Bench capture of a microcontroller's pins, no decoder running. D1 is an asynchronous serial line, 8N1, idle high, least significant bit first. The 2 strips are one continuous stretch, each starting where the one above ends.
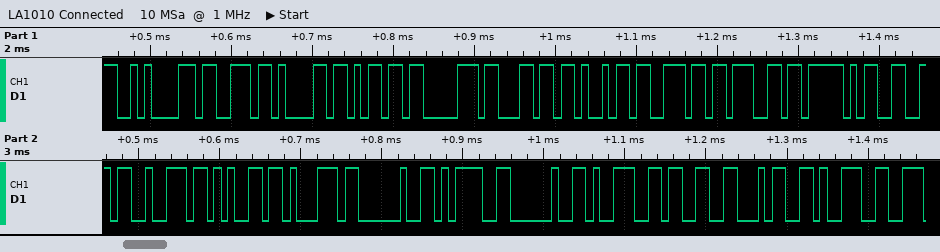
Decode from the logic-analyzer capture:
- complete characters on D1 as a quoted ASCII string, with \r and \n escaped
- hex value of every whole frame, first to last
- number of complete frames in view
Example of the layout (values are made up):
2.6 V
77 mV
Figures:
"\nsampling_freq = 9349"
0A 73 61 6D 70 6C 69 6E 67 5F 66 72 65 71 20 3D 20 39 33 34 39
21
